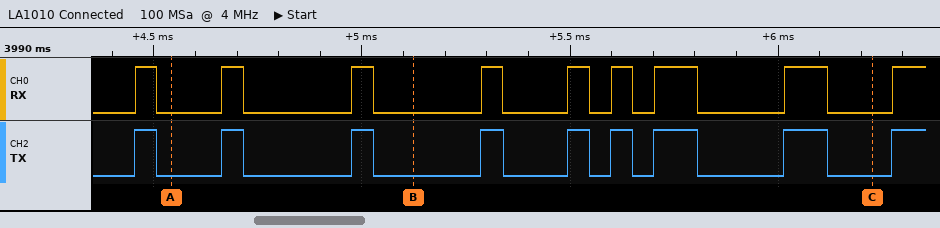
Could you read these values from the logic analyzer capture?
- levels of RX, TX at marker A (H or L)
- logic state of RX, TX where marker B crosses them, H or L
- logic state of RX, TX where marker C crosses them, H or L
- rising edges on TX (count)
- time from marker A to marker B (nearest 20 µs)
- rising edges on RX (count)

RX=L, TX=L
RX=L, TX=L
RX=L, TX=L
9
580 µs
9
